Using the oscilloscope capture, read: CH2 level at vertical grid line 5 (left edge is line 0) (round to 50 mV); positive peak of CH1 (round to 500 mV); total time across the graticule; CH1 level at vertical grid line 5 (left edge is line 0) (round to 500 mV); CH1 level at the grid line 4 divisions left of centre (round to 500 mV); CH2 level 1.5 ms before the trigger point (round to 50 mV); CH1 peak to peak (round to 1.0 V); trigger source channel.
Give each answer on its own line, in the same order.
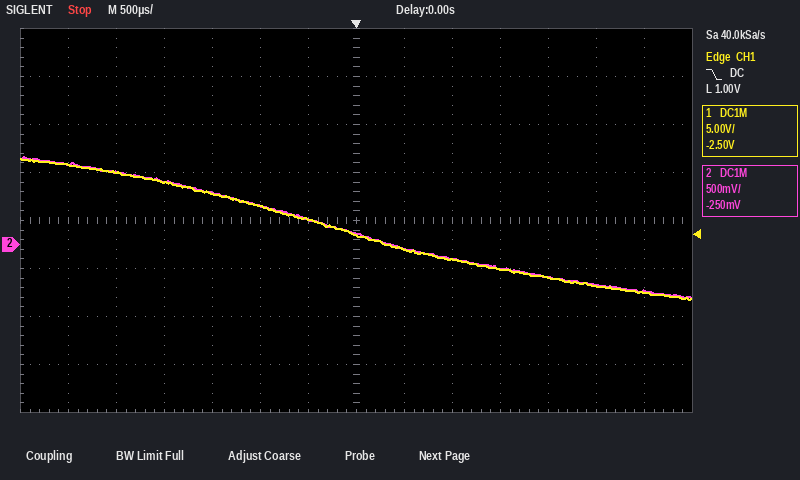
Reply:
400 mV
9.0 V
7 ms
4.0 V
6.5 V
550 mV
15.0 V
CH1
